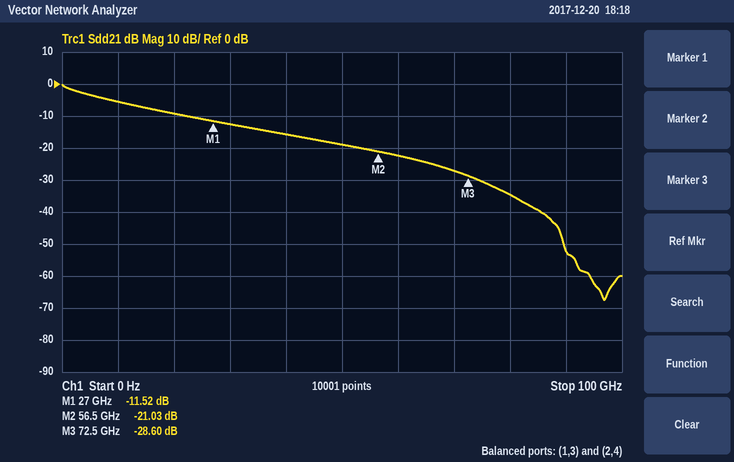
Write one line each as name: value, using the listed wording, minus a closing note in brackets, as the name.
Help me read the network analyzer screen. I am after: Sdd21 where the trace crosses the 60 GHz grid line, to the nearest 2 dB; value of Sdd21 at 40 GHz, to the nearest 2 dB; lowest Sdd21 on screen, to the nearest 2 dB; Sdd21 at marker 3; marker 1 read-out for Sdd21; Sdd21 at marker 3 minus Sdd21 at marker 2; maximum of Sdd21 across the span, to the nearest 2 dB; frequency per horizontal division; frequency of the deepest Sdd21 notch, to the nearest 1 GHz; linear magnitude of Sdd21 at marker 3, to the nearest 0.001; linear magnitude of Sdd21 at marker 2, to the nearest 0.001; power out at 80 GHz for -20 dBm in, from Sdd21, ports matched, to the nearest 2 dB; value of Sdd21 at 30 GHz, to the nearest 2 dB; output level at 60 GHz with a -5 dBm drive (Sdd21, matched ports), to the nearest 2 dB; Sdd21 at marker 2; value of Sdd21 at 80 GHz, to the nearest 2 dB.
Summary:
Sdd21 where the trace crosses the 60 GHz grid line, to the nearest 2 dB: -22 dB
value of Sdd21 at 40 GHz, to the nearest 2 dB: -16 dB
lowest Sdd21 on screen, to the nearest 2 dB: -68 dB
Sdd21 at marker 3: -28.60 dB
marker 1 read-out for Sdd21: -11.52 dB
Sdd21 at marker 3 minus Sdd21 at marker 2: -7.57 dB
maximum of Sdd21 across the span, to the nearest 2 dB: 0 dB
frequency per horizontal division: 10 GHz
frequency of the deepest Sdd21 notch, to the nearest 1 GHz: 97 GHz
linear magnitude of Sdd21 at marker 3, to the nearest 0.001: 0.037
linear magnitude of Sdd21 at marker 2, to the nearest 0.001: 0.089
power out at 80 GHz for -20 dBm in, from Sdd21, ports matched, to the nearest 2 dB: -54 dBm
value of Sdd21 at 30 GHz, to the nearest 2 dB: -12 dB
output level at 60 GHz with a -5 dBm drive (Sdd21, matched ports), to the nearest 2 dB: -28 dBm
Sdd21 at marker 2: -21.03 dB
value of Sdd21 at 80 GHz, to the nearest 2 dB: -34 dB
